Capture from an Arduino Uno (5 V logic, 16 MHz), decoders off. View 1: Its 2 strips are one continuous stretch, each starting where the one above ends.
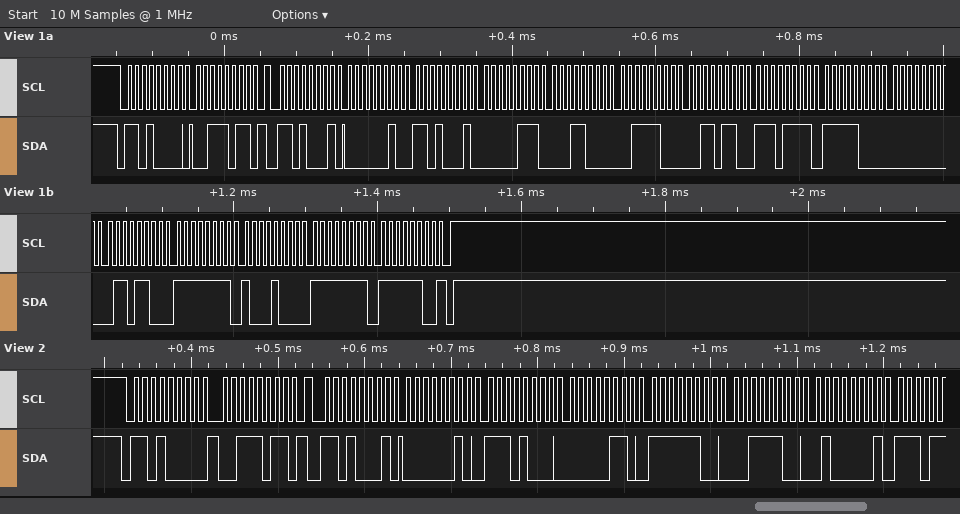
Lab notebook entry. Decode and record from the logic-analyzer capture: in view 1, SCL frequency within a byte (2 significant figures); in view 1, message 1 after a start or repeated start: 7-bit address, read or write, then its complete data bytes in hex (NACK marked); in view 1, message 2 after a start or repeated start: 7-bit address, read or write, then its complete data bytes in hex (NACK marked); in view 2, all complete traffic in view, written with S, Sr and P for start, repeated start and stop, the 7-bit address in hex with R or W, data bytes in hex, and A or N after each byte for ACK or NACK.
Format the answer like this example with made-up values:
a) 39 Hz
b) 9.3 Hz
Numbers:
a) 100 kHz
b) 0x68 write: 3B
c) 0x68 read: 02 D1 07 18 3C 36 EF F8 00 6C FF 88 FF FC NACK
d) S 68W A 3B A Sr 68R A 02 A E8 A 06 A FC A 3C A 41 A
